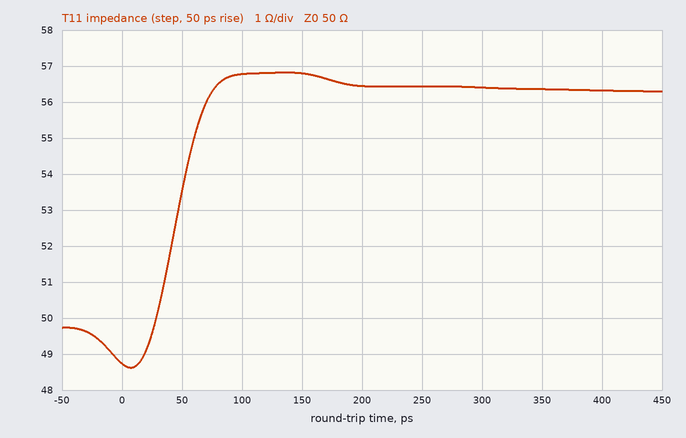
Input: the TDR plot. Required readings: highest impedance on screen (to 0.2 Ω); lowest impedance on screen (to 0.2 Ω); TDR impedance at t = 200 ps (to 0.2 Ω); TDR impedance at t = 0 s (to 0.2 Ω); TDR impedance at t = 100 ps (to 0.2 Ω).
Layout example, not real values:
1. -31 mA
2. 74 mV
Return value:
1. 56.8 Ω
2. 48.6 Ω
3. 56.4 Ω
4. 48.8 Ω
5. 56.8 Ω
